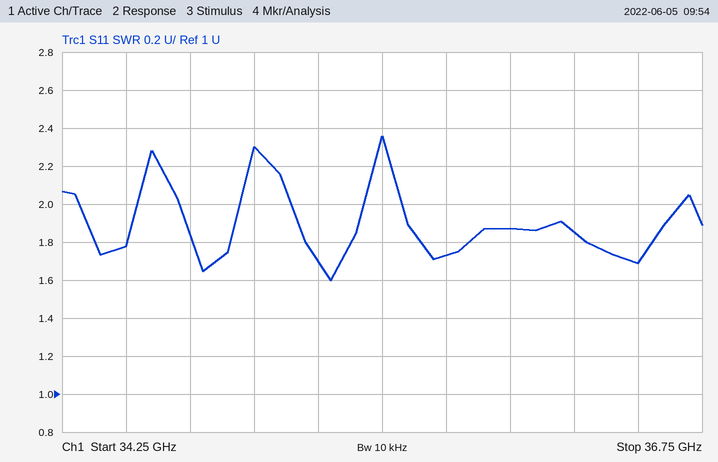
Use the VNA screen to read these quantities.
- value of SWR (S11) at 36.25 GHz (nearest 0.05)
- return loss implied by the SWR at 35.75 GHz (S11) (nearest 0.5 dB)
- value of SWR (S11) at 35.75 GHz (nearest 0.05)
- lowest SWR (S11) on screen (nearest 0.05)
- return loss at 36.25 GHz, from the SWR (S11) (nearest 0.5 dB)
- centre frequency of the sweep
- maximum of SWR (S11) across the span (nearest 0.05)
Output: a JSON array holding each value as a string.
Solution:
["1.85", "11.5 dB", "1.75", "1.60", "10.5 dB", "35.5 GHz", "2.35"]
